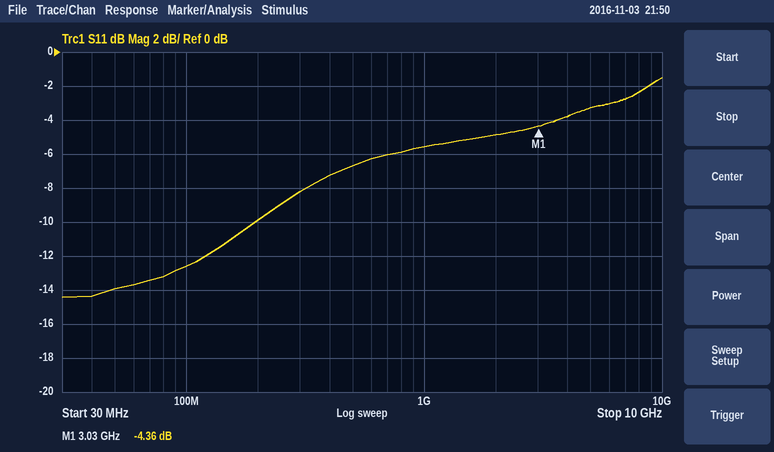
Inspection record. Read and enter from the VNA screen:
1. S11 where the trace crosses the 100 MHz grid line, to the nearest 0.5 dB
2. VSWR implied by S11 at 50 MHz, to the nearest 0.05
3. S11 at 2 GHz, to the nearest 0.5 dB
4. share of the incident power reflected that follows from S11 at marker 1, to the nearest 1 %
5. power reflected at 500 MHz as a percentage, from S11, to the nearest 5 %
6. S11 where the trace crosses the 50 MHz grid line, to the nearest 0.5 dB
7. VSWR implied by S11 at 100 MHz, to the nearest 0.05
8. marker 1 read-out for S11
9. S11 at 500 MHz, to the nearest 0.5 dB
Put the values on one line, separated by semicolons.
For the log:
-12.5 dB; 1.50; -5.0 dB; 37 %; 20 %; -14.0 dB; 1.60; -4.36 dB; -6.5 dB
